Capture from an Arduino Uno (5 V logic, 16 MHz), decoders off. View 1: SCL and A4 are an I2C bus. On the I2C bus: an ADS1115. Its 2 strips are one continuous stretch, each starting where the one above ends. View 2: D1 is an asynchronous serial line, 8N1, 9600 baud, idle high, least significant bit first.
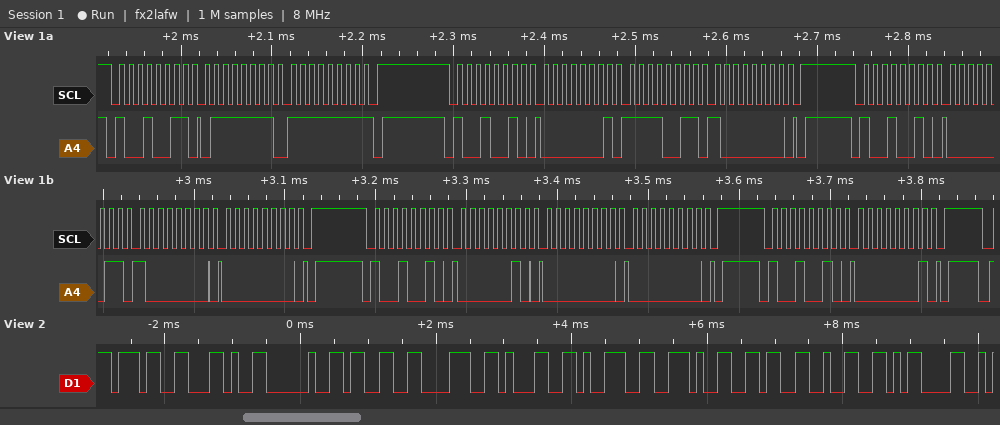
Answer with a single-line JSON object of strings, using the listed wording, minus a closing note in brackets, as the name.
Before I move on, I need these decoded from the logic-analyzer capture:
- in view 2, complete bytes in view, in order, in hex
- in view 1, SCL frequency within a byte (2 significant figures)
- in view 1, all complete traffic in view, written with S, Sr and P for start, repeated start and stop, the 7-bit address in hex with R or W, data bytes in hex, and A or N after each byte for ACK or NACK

{"in view 2, complete bytes in view, in order, in hex": "37 2C 20 33 38 31 39 2E 36 32 0D", "in view 1, SCL frequency within a byte": "100 kHz", "in view 1, all complete traffic in view, written with S, Sr and P for start, repeated start and stop, the 7-bit address in hex with R or W, data bytes in hex, and A or N after each byte for ACK or NACK": "S 49R A 7F A FF N P S 49W A 01 A F3 A 80 A P S 49W A 03 A 80 A 00 A P S 49W A 02 A 00 A 00 A P S 49W A 01 A P"}
